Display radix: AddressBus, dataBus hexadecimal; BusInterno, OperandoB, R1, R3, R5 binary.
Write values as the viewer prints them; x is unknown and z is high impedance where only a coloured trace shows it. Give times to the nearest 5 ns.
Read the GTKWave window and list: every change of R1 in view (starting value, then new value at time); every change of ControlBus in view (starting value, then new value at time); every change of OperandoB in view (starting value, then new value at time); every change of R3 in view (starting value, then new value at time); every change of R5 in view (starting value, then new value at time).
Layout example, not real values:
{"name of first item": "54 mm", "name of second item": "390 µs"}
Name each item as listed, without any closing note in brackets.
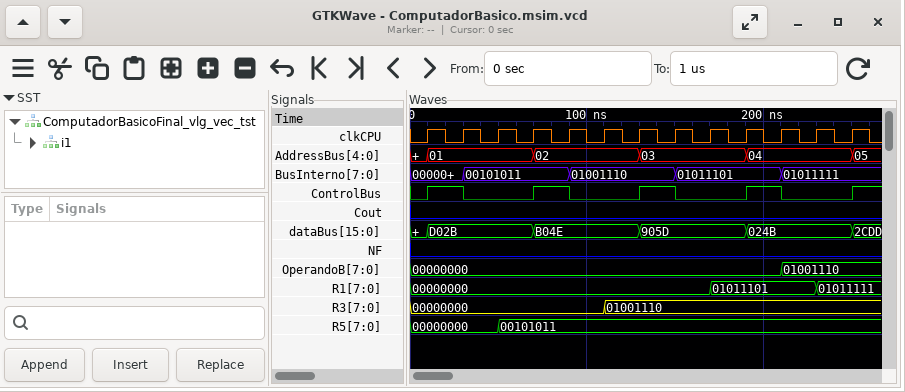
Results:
{"every change of R1 in view": "00000000, 01011101 at 170 ns, 01011111 at 230 ns", "every change of ControlBus in view": "0, 1 at 10 ns, 0 at 30 ns, 1 at 70 ns, 0 at 90 ns, 1 at 130 ns, 0 at 150 ns, 1 at 190 ns, 0 at 210 ns, 1 at 250 ns", "every change of OperandoB in view": "00000000, 01001110 at 210 ns", "every change of R3 in view": "00000000, 01001110 at 110 ns", "every change of R5 in view": "00000000, 00101011 at 50 ns"}
